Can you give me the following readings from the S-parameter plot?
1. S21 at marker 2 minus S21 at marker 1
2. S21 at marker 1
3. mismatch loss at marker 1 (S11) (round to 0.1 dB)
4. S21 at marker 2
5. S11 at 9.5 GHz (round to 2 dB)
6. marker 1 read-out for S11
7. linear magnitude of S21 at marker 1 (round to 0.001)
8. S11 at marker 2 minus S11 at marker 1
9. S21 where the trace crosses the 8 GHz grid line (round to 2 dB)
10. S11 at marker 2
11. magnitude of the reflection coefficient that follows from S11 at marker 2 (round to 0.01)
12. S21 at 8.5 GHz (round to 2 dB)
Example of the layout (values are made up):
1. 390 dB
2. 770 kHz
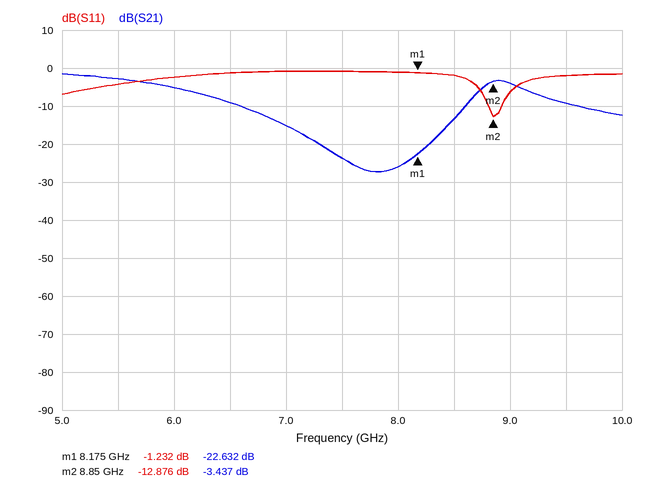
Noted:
1. 19.195 dB
2. -22.632 dB
3. 6.1 dB
4. -3.437 dB
5. -2 dB
6. -1.232 dB
7. 0.074
8. -11.644 dB
9. -26 dB
10. -12.876 dB
11. 0.23
12. -14 dB
